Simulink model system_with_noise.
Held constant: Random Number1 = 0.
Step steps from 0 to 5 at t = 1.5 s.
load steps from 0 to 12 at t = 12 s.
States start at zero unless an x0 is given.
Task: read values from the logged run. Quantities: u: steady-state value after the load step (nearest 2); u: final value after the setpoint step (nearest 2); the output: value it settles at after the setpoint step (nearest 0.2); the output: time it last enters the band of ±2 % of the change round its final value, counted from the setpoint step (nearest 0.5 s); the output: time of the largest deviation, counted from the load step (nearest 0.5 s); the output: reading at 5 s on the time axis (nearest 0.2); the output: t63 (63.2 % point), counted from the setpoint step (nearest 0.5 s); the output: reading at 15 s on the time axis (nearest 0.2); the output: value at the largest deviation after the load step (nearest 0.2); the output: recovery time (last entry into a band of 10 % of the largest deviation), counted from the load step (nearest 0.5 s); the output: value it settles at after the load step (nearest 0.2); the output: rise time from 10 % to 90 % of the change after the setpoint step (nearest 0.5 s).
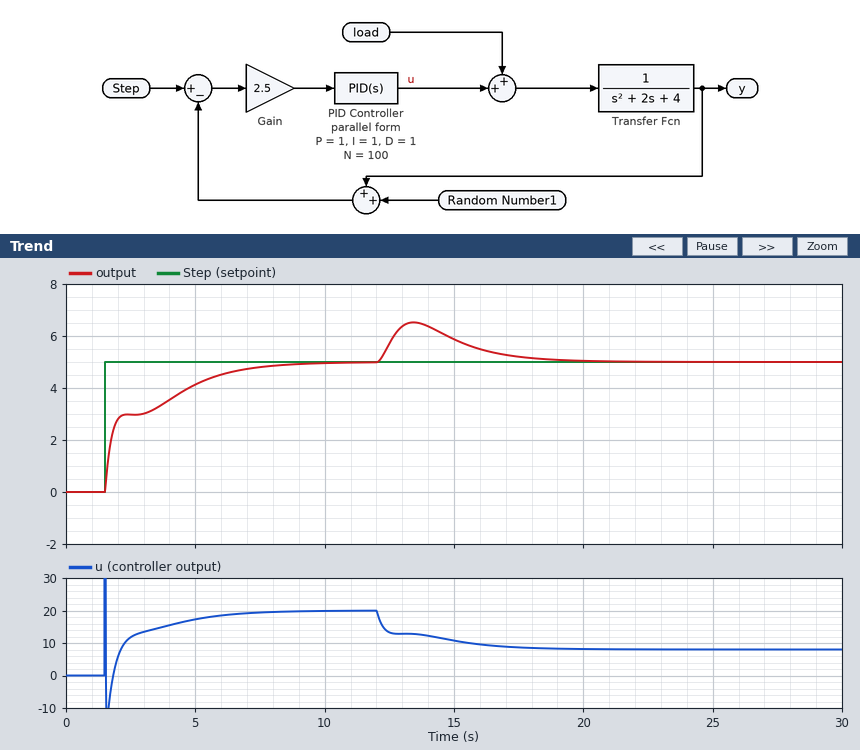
8
20
5.0
7.0 s
1.5 s
4.2
2.0 s
5.8
6.6
6.0 s
5.0
4.5 s
